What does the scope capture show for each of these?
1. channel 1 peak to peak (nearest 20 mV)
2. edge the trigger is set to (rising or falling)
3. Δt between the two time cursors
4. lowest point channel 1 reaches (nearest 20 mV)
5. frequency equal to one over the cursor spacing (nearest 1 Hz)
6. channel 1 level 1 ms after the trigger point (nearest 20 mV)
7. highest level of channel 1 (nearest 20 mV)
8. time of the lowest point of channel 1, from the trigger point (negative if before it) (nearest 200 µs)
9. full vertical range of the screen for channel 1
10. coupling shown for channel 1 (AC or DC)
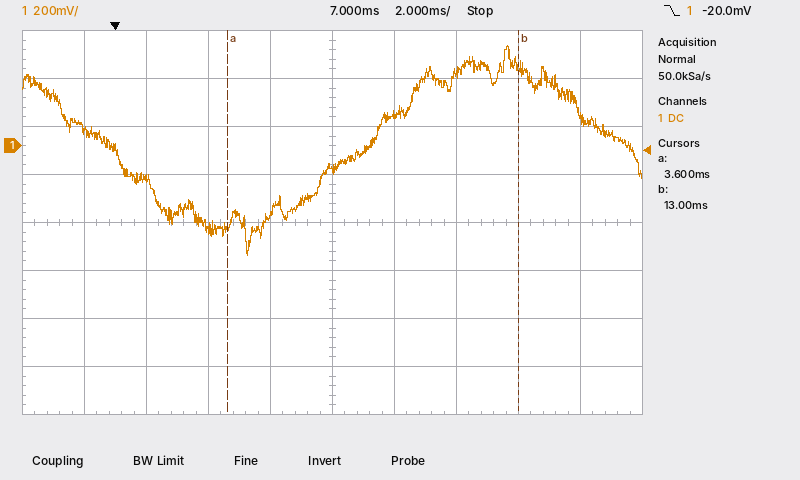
880 mV
falling
9.4 ms
-460 mV
106 Hz
-140 mV
420 mV
+4.2 ms
1.6 V
DC
